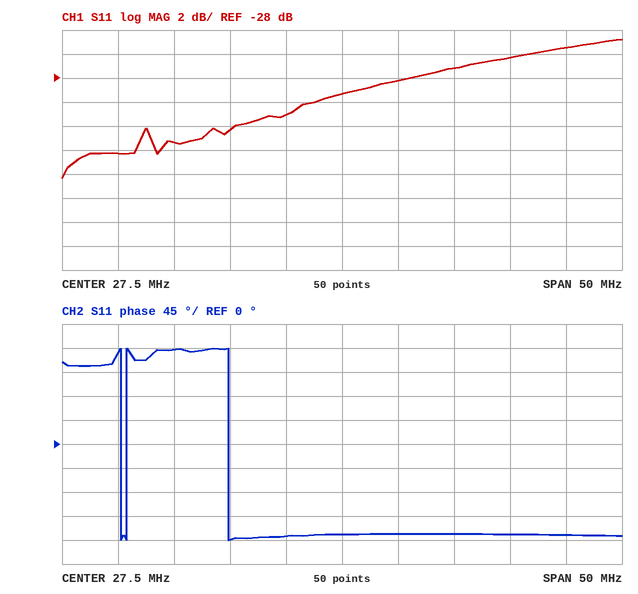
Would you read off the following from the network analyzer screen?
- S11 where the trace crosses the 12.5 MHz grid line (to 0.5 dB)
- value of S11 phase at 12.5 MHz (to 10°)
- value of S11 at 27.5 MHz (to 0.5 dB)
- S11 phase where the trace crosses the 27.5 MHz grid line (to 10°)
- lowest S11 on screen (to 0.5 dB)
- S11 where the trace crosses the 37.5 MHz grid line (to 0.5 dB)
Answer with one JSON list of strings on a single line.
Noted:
["-33.5 dB", "180°", "-29.5 dB", "-170°", "-36.5 dB", "-27.0 dB"]
